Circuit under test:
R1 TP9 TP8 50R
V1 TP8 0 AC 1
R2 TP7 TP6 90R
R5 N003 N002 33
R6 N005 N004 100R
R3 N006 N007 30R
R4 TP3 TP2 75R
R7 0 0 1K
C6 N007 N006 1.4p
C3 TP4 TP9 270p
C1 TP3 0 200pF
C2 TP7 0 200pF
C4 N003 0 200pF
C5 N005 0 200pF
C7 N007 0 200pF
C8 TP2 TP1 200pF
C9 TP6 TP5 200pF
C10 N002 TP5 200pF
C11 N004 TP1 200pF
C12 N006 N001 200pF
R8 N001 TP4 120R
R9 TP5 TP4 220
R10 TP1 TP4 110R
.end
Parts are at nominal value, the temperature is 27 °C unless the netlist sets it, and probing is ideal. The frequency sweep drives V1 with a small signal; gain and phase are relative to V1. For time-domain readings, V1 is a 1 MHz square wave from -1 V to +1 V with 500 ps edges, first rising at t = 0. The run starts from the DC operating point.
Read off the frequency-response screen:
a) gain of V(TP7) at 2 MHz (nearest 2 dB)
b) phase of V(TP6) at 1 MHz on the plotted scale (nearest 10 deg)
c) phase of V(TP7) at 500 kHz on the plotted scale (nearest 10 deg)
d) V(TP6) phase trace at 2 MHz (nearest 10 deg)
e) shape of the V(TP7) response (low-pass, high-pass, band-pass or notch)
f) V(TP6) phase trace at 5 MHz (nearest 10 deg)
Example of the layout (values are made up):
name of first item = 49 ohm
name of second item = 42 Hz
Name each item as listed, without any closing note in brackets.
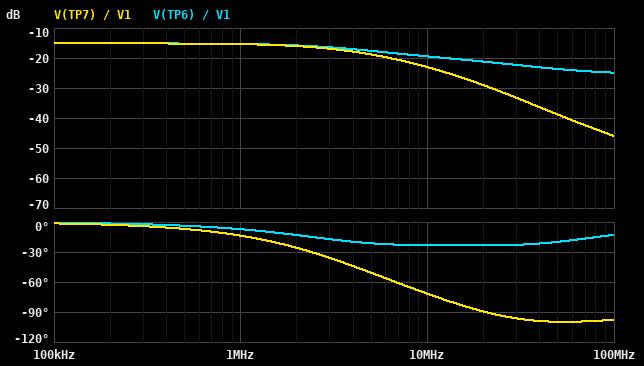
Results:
gain of V(TP7) at 2 MHz = -16 dB
phase of V(TP6) at 1 MHz on the plotted scale = -10 deg
phase of V(TP7) at 500 kHz on the plotted scale = -10 deg
V(TP6) phase trace at 2 MHz = -10 deg
shape of the V(TP7) response = low-pass
V(TP6) phase trace at 5 MHz = -20 deg
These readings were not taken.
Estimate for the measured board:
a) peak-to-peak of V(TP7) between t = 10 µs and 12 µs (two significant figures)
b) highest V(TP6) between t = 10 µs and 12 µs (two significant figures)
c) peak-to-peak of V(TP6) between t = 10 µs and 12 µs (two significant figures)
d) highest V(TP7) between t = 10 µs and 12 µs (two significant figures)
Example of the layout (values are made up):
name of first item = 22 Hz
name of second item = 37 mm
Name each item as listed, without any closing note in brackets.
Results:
peak-to-peak of V(TP7) between t = 10 µs and 12 µs = 350 mV
highest V(TP6) between t = 10 µs and 12 µs = 350 mV
peak-to-peak of V(TP6) between t = 10 µs and 12 µs = 350 mV
highest V(TP7) between t = 10 µs and 12 µs = 350 mV
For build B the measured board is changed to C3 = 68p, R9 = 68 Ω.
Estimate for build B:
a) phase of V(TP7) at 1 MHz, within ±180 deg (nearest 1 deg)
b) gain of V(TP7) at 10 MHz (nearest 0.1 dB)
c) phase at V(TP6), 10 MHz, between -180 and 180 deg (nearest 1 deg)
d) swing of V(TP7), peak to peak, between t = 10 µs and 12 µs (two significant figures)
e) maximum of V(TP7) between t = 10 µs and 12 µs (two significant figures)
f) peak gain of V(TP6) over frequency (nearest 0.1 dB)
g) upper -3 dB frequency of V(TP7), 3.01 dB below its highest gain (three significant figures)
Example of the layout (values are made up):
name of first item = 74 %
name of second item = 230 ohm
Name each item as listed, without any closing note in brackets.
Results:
phase of V(TP7) at 1 MHz, within ±180 deg = -2 deg
gain of V(TP7) at 10 MHz = -24.7 dB
phase at V(TP6), 10 MHz, between -180 and 180 deg = 22 deg
swing of V(TP7), peak to peak, between t = 10 µs and 12 µs = 130 mV
maximum of V(TP7) between t = 10 µs and 12 µs = 120 mV
peak gain of V(TP6) over frequency = -17.9 dB
upper -3 dB frequency of V(TP7), 3.01 dB below its highest gain = 22.0 MHz
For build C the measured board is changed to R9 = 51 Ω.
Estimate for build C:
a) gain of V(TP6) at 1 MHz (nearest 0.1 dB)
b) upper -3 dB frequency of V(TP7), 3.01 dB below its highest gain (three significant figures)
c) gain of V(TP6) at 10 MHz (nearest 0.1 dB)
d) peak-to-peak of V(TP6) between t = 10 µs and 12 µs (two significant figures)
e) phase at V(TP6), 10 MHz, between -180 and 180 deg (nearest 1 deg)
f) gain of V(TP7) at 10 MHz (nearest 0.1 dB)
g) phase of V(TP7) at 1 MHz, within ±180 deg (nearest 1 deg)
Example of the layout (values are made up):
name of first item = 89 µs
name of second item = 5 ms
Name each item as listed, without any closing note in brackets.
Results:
gain of V(TP6) at 1 MHz = -15.1 dB
upper -3 dB frequency of V(TP7), 3.01 dB below its highest gain = 11.6 MHz
gain of V(TP6) at 10 MHz = -13.8 dB
peak-to-peak of V(TP6) between t = 10 µs and 12 µs = 450 mV
phase at V(TP6), 10 MHz, between -180 and 180 deg = 0 deg
gain of V(TP7) at 10 MHz = -17.4 dB
phase of V(TP7) at 1 MHz, within ±180 deg = -5 deg
